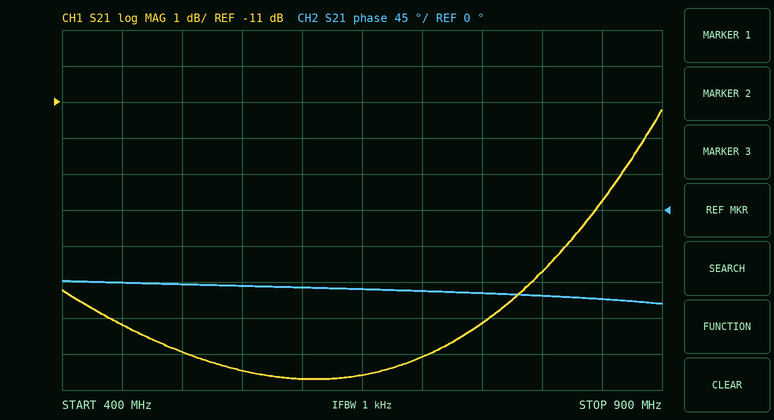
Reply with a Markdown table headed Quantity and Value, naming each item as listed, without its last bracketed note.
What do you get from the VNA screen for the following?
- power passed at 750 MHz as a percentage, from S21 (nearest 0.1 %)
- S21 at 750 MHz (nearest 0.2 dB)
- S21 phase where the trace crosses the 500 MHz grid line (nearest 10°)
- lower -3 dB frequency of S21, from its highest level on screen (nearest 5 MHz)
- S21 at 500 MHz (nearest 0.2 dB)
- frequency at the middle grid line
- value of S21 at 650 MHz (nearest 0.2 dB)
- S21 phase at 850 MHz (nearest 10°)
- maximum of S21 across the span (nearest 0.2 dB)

| Quantity | Value |
|---|---|
| power passed at 750 MHz as a percentage, from S21 | 1.9 % |
| S21 at 750 MHz | -17.2 dB |
| S21 phase where the trace crosses the 500 MHz grid line | -90° |
| lower -3 dB frequency of S21, from its highest level on screen | 840 MHz |
| S21 at 500 MHz | -18.0 dB |
| frequency at the middle grid line | 650 MHz |
| value of S21 at 650 MHz | -18.6 dB |
| S21 phase at 850 MHz | -110° |
| maximum of S21 across the span | -11.2 dB |
